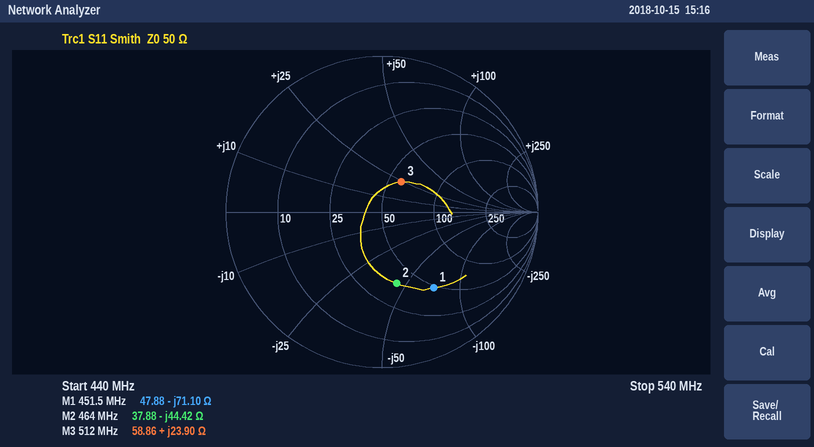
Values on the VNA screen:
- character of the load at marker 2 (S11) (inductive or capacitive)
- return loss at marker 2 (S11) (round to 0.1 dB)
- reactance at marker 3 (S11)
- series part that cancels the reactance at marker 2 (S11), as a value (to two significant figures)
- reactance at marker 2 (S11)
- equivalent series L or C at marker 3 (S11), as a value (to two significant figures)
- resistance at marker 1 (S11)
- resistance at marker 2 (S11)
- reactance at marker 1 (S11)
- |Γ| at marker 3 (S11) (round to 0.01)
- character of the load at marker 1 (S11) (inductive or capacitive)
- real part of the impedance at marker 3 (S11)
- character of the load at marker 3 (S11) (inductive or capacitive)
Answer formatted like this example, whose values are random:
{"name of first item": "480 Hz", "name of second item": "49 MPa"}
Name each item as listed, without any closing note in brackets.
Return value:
{"character of the load at marker 2 (S11)": "capacitive", "return loss at marker 2 (S11)": "6.6 dB", "reactance at marker 3": "+23.90 Ω", "series part that cancels the reactance at marker 2 (S11), as a value": "15 nH", "reactance at marker 2": "-44.42 Ω", "equivalent series L or C at marker 3 (S11), as a value": "7.4 nH", "resistance at marker 1": "47.88 Ω", "resistance at marker 2": "37.88 Ω", "reactance at marker 1": "-71.10 Ω", "|Γ| at marker 3 (S11)": "0.23", "character of the load at marker 1 (S11)": "capacitive", "real part of the impedance at marker 3": "58.86 Ω", "character of the load at marker 3 (S11)": "inductive"}
